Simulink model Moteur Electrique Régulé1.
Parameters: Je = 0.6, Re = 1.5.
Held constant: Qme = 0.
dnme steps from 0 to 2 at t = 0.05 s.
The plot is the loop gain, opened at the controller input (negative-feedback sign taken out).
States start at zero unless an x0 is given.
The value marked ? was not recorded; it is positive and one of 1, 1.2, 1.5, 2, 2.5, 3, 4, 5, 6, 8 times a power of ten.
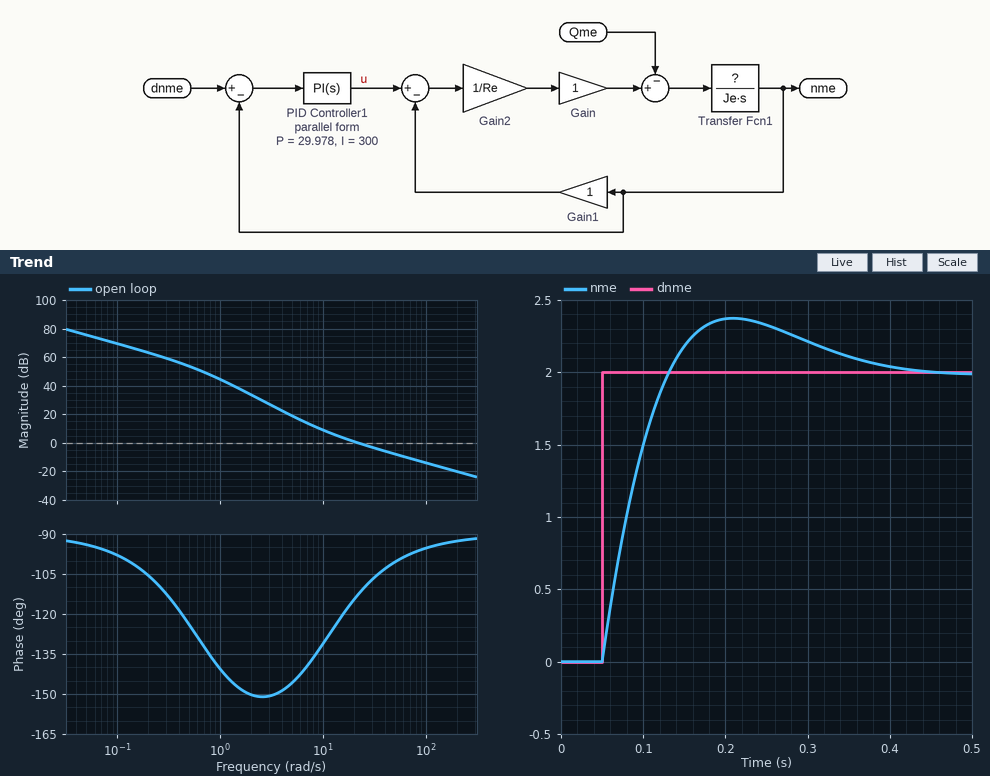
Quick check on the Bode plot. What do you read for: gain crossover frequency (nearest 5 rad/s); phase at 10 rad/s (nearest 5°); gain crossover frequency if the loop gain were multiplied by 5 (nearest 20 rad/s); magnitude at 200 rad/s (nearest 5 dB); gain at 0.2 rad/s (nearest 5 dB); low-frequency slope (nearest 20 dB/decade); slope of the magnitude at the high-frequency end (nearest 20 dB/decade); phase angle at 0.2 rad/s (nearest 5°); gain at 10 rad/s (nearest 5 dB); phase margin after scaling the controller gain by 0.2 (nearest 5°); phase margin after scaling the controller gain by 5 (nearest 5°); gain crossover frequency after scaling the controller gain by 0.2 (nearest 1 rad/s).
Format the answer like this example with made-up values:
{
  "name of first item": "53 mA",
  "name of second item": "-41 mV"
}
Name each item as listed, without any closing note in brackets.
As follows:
{
  "gain crossover frequency": "20 rad/s",
  "phase at 10 rad/s": "-130°",
  "gain crossover frequency if the loop gain were multiplied by 5": "100 rad/s",
  "magnitude at 200 rad/s": "-20 dB",
  "gain at 0.2 rad/s": "65 dB",
  "low-frequency slope": "-20 dB/decade",
  "slope of the magnitude at the high-frequency end": "-20 dB/decade",
  "phase angle at 0.2 rad/s": "-105°",
  "gain at 10 rad/s": "10 dB",
  "phase margin after scaling the controller gain by 0.2": "40°",
  "phase margin after scaling the controller gain by 5": "85°",
  "gain crossover frequency after scaling the controller gain by 0.2": "7 rad/s"
}
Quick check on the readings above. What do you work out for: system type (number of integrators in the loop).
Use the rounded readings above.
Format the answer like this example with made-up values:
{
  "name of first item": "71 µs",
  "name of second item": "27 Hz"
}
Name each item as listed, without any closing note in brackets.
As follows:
{
  "system type": "1"
}
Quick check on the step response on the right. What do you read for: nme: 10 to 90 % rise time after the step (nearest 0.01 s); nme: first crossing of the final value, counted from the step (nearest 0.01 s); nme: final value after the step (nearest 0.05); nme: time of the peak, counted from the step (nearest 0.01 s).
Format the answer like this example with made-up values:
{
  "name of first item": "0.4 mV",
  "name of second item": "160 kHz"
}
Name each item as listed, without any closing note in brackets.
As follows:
{
  "nme: 10 to 90 % rise time after the step": "0.06 s",
  "nme: first crossing of the final value, counted from the step": "0.08 s",
  "nme: final value after the step": "2.00",
  "nme: time of the peak, counted from the step": "0.16 s"
}
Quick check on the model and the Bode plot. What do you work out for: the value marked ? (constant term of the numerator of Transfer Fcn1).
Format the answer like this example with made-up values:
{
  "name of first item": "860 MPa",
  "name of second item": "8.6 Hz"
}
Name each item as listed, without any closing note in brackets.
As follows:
{
  "the value marked ?": "0.6"
}
